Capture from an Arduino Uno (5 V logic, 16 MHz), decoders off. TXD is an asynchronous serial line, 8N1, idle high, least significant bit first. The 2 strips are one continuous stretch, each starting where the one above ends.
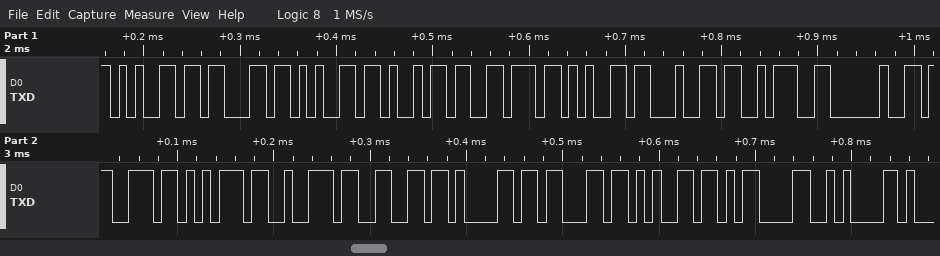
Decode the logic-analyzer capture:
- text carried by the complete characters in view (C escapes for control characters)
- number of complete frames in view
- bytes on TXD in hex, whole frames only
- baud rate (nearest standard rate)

"eceived: surface\r\n"
18
0x65 0x63 0x65 0x69 0x76 0x65 0x64 0x3A 0x20 0x73 0x75 0x72 0x66 0x61 0x63 0x65 0x0D 0x0A
115200 baud
